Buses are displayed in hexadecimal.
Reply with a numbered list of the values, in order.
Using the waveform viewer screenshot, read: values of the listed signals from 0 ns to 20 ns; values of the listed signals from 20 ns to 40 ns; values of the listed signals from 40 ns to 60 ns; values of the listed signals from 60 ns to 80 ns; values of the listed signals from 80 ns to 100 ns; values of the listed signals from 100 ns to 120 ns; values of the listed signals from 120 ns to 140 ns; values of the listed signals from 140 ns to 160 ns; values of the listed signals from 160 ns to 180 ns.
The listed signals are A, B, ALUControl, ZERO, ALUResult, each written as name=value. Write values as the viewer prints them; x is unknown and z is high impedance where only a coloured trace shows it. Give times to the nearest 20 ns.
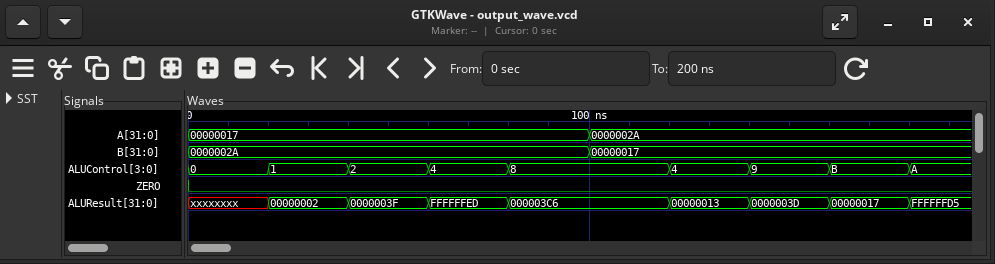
1. A=00000017, B=0000002A, ALUControl=0, ZERO=0, ALUResult=xxxxxxxx
2. A=00000017, B=0000002A, ALUControl=1, ZERO=0, ALUResult=00000002
3. A=00000017, B=0000002A, ALUControl=2, ZERO=0, ALUResult=0000003F
4. A=00000017, B=0000002A, ALUControl=4, ZERO=0, ALUResult=FFFFFFED
5. A=00000017, B=0000002A, ALUControl=8, ZERO=0, ALUResult=000003C6
6. A=0000002A, B=00000017, ALUControl=8, ZERO=0, ALUResult=000003C6
7. A=0000002A, B=00000017, ALUControl=4, ZERO=0, ALUResult=00000013
8. A=0000002A, B=00000017, ALUControl=9, ZERO=0, ALUResult=0000003D
9. A=0000002A, B=00000017, ALUControl=B, ZERO=0, ALUResult=00000017
